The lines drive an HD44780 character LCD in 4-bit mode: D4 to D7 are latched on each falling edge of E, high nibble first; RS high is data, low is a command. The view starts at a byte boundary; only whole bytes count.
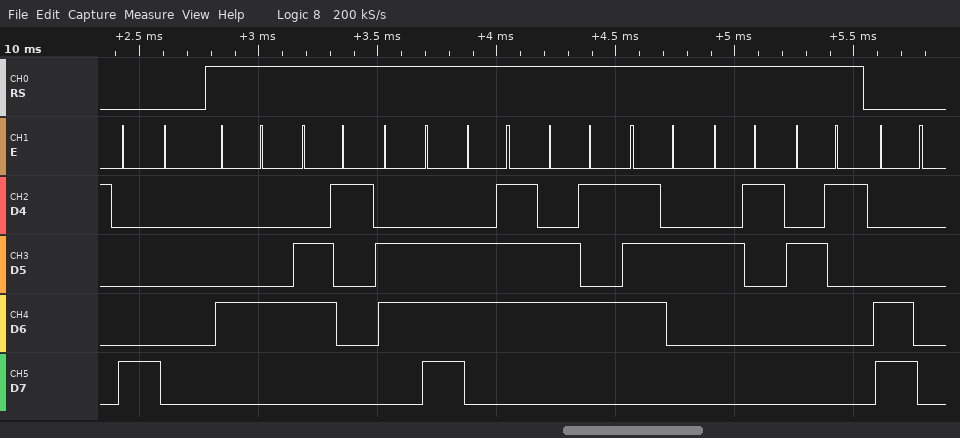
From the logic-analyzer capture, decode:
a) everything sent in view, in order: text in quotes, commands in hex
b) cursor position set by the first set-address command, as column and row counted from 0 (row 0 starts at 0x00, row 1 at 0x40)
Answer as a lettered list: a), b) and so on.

a) 0x80 "Danger!!" 0xC0
b) column 0, row 0
